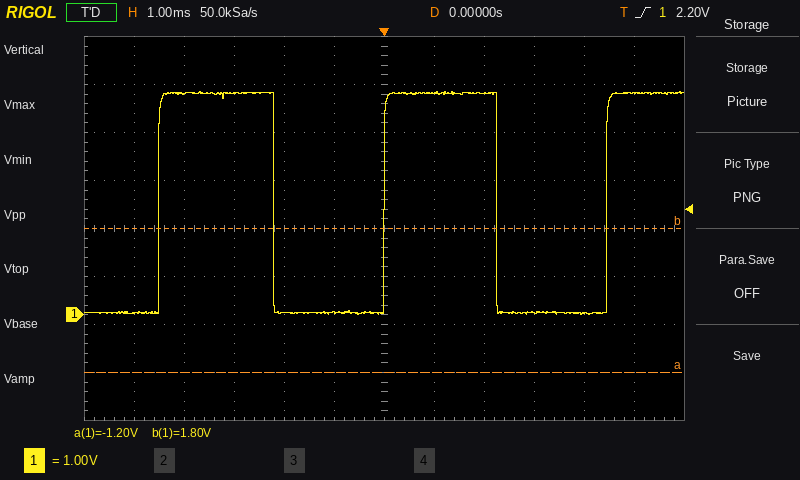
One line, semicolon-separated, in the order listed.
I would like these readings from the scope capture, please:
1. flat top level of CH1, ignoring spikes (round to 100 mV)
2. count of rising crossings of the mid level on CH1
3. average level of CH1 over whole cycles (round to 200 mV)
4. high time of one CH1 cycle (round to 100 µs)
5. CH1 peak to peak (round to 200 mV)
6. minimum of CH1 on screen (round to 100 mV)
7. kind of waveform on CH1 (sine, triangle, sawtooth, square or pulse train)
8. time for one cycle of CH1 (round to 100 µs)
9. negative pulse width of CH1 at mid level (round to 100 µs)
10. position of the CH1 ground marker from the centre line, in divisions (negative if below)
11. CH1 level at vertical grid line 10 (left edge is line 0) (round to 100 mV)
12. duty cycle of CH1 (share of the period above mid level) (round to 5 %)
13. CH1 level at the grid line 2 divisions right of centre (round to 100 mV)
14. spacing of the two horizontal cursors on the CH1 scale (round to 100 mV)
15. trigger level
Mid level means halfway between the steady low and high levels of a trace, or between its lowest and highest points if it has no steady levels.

4.6 V; 3; 2.4 V; 2.3 ms; 4.6 V; 0.0 V; square; 4.5 ms; 2.2 ms; -1.8 div; 0.0 V; 50 %; 4.6 V; 3.0 V; 2.20 V
